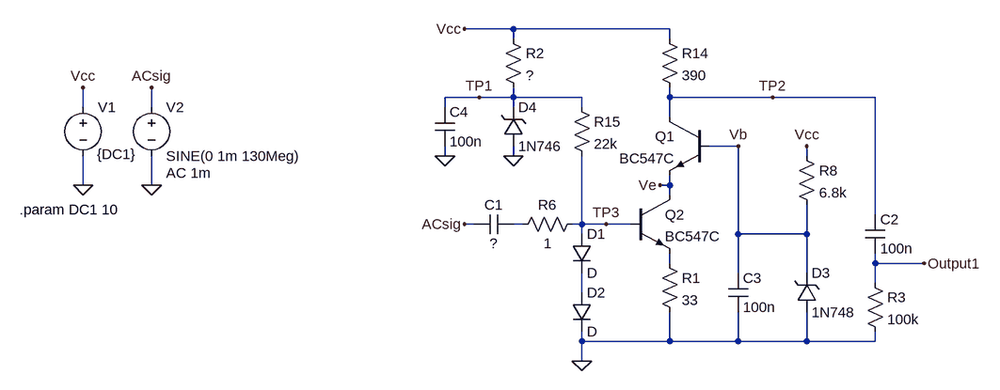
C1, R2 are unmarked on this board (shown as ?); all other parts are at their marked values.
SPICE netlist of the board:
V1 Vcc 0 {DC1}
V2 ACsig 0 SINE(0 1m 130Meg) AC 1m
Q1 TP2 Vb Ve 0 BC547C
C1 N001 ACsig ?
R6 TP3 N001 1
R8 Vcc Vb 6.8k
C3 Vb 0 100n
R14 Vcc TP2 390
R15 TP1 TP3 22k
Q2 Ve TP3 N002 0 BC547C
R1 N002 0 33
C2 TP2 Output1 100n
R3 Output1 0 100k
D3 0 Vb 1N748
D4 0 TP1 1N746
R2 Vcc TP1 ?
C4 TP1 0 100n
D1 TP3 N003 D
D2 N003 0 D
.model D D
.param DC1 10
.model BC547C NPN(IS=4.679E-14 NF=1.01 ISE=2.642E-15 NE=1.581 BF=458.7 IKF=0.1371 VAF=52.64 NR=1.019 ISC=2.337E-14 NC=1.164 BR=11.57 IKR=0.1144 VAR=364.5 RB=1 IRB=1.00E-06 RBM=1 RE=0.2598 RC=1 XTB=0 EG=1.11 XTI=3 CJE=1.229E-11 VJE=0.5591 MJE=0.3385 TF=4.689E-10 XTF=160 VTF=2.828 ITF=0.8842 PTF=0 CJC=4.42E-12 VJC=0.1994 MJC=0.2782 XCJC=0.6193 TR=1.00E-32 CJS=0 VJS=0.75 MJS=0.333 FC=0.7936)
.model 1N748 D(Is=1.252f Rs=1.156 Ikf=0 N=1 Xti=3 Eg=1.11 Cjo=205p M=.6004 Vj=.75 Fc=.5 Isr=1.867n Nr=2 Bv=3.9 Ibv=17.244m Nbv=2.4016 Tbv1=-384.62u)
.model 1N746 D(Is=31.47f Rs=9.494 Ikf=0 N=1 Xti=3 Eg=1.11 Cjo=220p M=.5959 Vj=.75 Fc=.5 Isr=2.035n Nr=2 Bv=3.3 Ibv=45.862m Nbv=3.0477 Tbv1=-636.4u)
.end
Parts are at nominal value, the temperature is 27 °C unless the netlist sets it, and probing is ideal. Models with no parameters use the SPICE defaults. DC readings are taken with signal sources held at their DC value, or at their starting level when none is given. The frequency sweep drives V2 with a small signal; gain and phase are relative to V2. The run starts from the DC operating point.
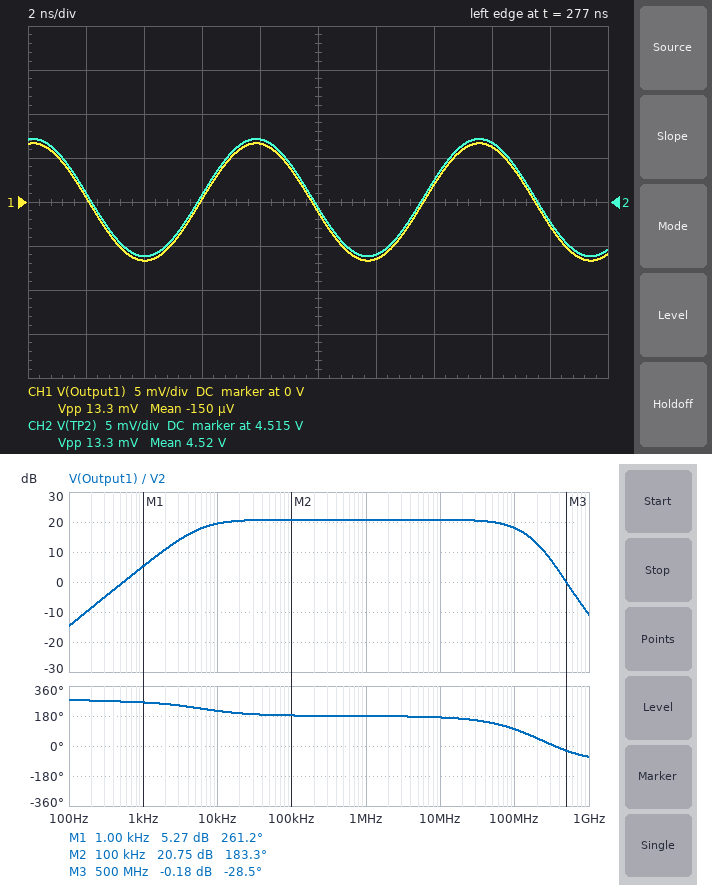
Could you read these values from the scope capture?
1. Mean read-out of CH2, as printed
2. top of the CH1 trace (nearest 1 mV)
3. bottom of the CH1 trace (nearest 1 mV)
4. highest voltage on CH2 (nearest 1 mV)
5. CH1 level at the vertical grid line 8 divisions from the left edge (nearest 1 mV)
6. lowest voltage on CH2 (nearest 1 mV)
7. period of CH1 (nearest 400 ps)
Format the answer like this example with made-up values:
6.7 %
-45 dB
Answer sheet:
4.52 V
7 mV
-7 mV
4.522 V
6 mV
4.509 V
7.6 ns
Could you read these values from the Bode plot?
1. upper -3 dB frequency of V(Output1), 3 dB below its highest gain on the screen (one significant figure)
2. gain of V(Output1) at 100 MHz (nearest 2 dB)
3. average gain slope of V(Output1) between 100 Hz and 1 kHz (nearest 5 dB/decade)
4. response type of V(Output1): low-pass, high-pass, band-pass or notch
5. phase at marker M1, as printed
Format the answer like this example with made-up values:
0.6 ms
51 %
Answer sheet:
100 MHz
18 dB
20 dB/decade
band-pass
261.2 deg
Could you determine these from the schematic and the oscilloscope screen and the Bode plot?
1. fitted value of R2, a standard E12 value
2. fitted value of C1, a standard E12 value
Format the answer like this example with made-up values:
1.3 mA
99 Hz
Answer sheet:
1.8 kΩ
33 nF
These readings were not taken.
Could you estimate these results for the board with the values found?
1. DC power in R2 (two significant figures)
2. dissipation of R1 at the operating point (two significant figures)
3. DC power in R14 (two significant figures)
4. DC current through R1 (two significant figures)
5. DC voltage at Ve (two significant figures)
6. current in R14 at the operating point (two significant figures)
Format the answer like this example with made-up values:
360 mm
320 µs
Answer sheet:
26 mW
6.6 mW
77 mW
14 mA
3.0 V
14 mA
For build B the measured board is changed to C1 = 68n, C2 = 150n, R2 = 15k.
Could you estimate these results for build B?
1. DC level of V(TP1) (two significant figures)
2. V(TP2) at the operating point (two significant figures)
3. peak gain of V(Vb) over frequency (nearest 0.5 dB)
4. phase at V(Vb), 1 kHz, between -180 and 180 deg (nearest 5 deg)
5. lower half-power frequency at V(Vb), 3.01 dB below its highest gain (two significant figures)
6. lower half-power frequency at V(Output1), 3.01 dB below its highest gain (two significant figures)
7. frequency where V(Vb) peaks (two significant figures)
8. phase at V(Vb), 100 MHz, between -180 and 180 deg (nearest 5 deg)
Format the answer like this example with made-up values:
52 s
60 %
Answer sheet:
2.9 V
4.6 V
-46.0 dB
-115 deg
2.1 kHz
2.5 kHz
7.5 kHz
115 deg
